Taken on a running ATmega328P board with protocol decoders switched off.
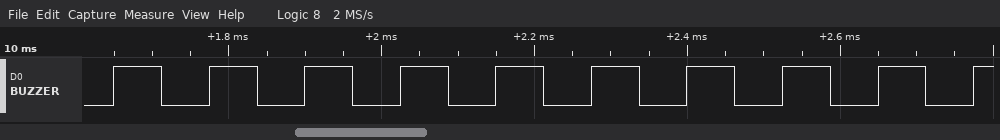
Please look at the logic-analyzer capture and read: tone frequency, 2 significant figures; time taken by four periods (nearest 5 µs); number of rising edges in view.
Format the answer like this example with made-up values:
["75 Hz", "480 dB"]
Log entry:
["8.0 kHz", "500 µs", "10"]
